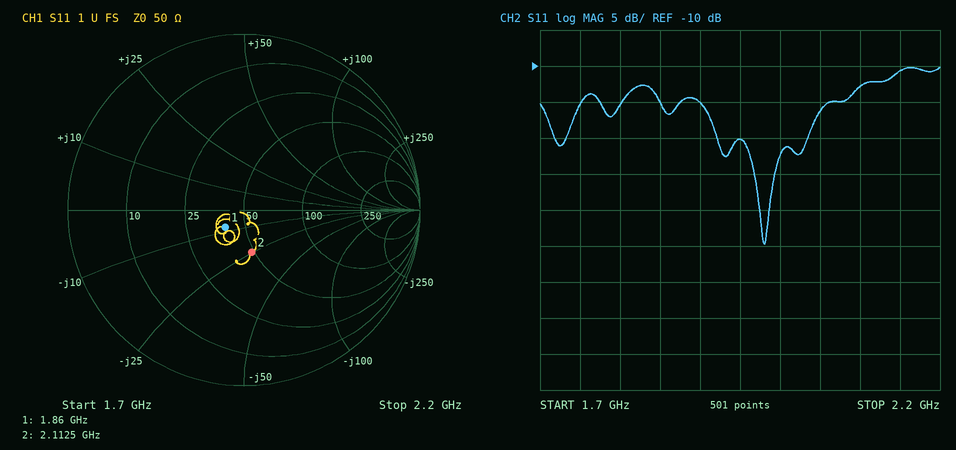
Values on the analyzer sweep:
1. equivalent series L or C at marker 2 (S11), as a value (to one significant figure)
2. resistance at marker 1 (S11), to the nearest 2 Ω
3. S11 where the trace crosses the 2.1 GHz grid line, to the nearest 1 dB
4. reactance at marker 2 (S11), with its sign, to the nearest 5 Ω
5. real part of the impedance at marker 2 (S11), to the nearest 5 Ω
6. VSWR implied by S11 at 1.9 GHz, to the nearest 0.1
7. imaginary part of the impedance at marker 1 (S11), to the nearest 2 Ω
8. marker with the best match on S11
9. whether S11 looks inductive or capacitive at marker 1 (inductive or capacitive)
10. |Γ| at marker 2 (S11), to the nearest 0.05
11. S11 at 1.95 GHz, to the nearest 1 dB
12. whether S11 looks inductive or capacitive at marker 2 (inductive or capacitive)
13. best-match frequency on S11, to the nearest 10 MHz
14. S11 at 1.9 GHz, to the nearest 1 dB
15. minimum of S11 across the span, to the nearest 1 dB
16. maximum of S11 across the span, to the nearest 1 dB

3 pF
40 Ω
-13 dB
-25 Ω
50 Ω
1.4
-8 Ω
marker 1
capacitive
0.25
-20 dB
capacitive
1.98 GHz
-15 dB
-35 dB
-10 dB
